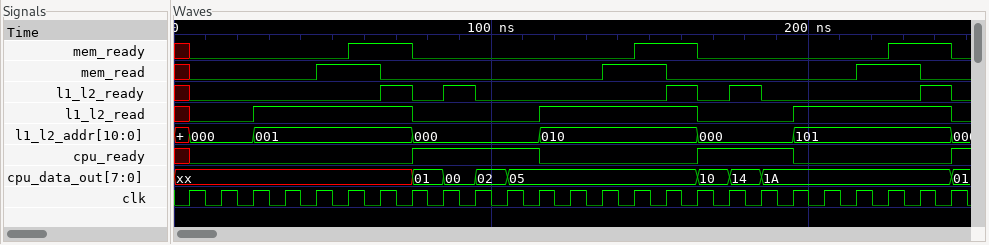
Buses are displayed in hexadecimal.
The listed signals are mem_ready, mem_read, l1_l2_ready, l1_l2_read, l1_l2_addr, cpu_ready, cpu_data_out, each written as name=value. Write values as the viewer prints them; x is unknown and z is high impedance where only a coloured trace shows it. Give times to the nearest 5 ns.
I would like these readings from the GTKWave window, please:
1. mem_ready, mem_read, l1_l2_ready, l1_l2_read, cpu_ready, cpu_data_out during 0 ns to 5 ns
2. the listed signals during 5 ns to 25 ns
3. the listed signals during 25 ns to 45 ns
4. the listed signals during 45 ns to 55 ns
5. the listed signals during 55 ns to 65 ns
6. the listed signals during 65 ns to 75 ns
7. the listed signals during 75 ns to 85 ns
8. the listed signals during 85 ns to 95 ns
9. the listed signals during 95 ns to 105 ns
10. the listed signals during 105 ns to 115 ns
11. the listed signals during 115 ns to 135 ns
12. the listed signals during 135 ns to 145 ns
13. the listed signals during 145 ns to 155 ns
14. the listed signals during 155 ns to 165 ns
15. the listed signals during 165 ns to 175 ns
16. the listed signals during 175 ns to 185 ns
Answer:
mem_ready=x, mem_read=x, l1_l2_ready=x, l1_l2_read=x, cpu_ready=x, cpu_data_out=xx
mem_ready=0, mem_read=0, l1_l2_ready=0, l1_l2_read=0, l1_l2_addr=000, cpu_ready=0, cpu_data_out=xx
mem_ready=0, mem_read=0, l1_l2_ready=0, l1_l2_read=1, l1_l2_addr=001, cpu_ready=0, cpu_data_out=xx
mem_ready=0, mem_read=1, l1_l2_ready=0, l1_l2_read=1, l1_l2_addr=001, cpu_ready=0, cpu_data_out=xx
mem_ready=1, mem_read=1, l1_l2_ready=0, l1_l2_read=1, l1_l2_addr=001, cpu_ready=0, cpu_data_out=xx
mem_ready=1, mem_read=0, l1_l2_ready=1, l1_l2_read=1, l1_l2_addr=001, cpu_ready=0, cpu_data_out=xx
mem_ready=0, mem_read=0, l1_l2_ready=0, l1_l2_read=0, l1_l2_addr=000, cpu_ready=1, cpu_data_out=01
mem_ready=0, mem_read=0, l1_l2_ready=1, l1_l2_read=0, l1_l2_addr=000, cpu_ready=1, cpu_data_out=00
mem_ready=0, mem_read=0, l1_l2_ready=0, l1_l2_read=0, l1_l2_addr=000, cpu_ready=1, cpu_data_out=02
mem_ready=0, mem_read=0, l1_l2_ready=0, l1_l2_read=0, l1_l2_addr=000, cpu_ready=1, cpu_data_out=05
mem_ready=0, mem_read=0, l1_l2_ready=0, l1_l2_read=1, l1_l2_addr=010, cpu_ready=0, cpu_data_out=05
mem_ready=0, mem_read=1, l1_l2_ready=0, l1_l2_read=1, l1_l2_addr=010, cpu_ready=0, cpu_data_out=05
mem_ready=1, mem_read=1, l1_l2_ready=0, l1_l2_read=1, l1_l2_addr=010, cpu_ready=0, cpu_data_out=05
mem_ready=1, mem_read=0, l1_l2_ready=1, l1_l2_read=1, l1_l2_addr=010, cpu_ready=0, cpu_data_out=05
mem_ready=0, mem_read=0, l1_l2_ready=0, l1_l2_read=0, l1_l2_addr=000, cpu_ready=1, cpu_data_out=10
mem_ready=0, mem_read=0, l1_l2_ready=1, l1_l2_read=0, l1_l2_addr=000, cpu_ready=1, cpu_data_out=14
